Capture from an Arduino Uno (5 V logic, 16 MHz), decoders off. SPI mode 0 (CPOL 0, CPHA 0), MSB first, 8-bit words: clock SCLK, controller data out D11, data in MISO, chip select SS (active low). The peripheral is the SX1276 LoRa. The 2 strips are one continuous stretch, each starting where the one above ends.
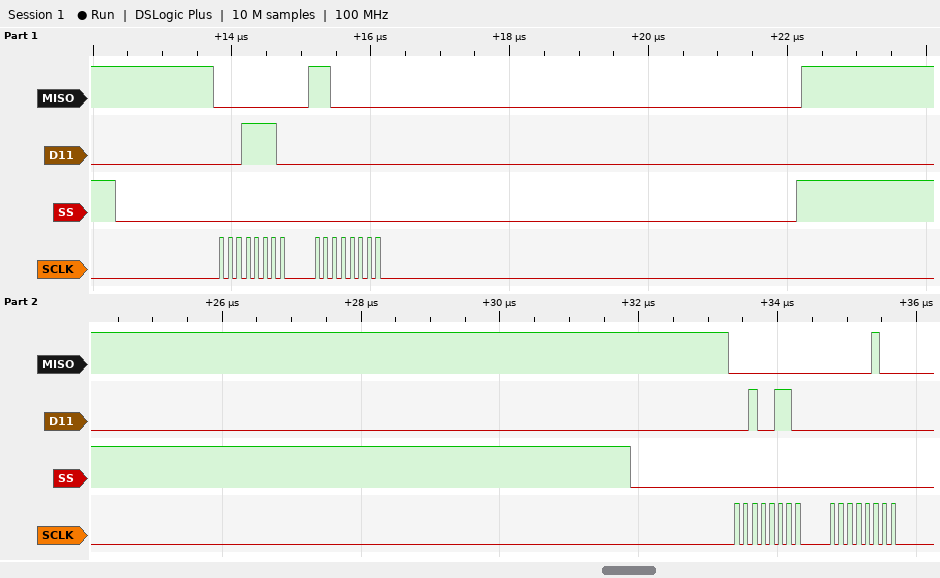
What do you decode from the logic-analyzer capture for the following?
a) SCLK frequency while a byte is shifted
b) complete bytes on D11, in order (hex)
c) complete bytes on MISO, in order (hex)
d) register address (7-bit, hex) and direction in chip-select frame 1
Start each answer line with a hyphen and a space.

- 8 MHz
- 1E 00 26 00
- 00 C0 00 04
- 0x1E read
